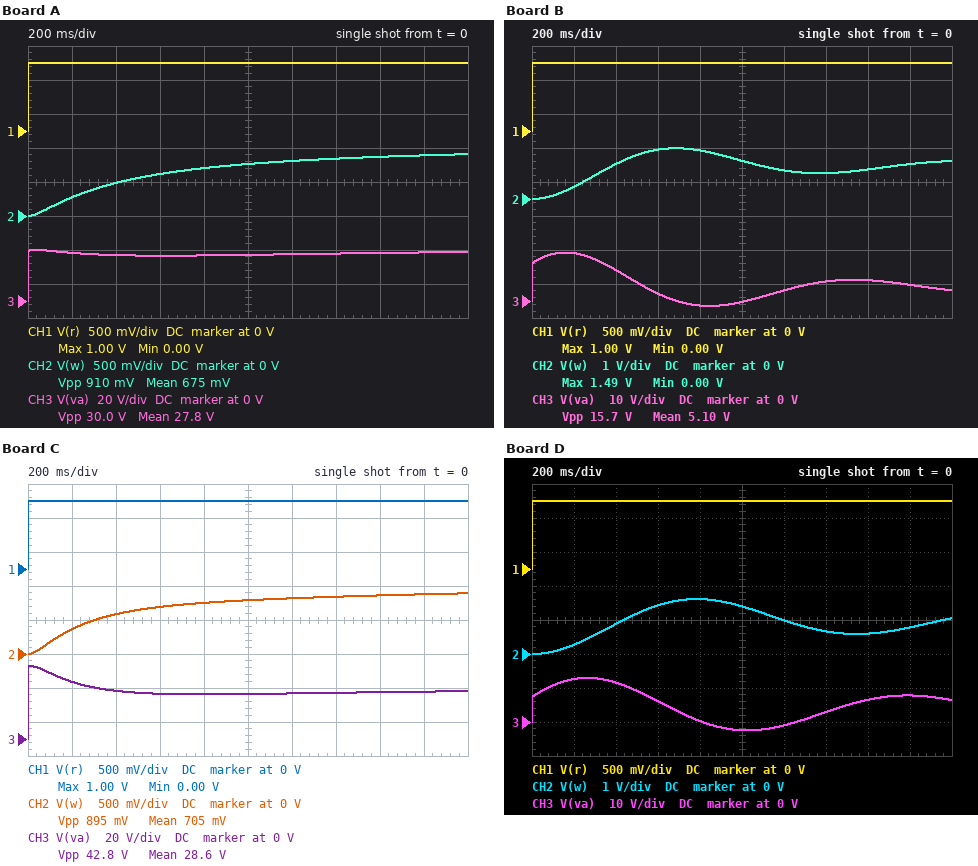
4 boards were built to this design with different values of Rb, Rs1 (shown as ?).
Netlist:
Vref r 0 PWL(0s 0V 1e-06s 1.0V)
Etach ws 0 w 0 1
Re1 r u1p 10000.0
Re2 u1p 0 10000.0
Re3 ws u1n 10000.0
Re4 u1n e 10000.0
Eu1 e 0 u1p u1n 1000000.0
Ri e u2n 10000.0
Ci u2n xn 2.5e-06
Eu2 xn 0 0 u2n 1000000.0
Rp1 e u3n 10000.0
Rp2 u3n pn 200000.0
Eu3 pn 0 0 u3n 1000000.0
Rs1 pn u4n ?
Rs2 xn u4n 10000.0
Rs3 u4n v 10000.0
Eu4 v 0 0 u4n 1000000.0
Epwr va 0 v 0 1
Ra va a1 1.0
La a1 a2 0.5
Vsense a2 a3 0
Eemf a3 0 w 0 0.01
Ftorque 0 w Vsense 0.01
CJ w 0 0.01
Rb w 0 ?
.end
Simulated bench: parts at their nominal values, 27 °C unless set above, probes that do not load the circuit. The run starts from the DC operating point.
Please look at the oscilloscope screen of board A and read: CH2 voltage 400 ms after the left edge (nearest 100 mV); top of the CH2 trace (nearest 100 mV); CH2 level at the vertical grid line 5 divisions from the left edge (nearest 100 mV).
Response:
500 mV
900 mV
800 mV
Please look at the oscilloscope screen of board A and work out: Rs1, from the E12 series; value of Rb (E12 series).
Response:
6.8 kΩ
3.3 Ω
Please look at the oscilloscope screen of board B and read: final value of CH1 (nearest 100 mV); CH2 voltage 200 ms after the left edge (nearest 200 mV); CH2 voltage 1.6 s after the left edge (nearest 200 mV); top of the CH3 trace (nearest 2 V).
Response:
1.0 V
400 mV
800 mV
14 V
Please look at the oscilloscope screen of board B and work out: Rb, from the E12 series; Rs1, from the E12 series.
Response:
27 Ω
18 kΩ
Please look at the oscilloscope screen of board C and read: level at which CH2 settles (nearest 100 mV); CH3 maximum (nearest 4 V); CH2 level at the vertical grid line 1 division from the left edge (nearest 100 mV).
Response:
900 mV
44 V
400 mV
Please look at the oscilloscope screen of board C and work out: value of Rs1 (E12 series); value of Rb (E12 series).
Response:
4.7 kΩ
3.3 Ω
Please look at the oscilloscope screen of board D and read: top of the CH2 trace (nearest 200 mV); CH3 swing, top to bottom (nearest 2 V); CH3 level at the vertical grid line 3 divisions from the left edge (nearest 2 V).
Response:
1.6 V
16 V
6 V
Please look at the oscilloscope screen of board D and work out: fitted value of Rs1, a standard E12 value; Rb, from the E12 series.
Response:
27 kΩ
27 Ω
